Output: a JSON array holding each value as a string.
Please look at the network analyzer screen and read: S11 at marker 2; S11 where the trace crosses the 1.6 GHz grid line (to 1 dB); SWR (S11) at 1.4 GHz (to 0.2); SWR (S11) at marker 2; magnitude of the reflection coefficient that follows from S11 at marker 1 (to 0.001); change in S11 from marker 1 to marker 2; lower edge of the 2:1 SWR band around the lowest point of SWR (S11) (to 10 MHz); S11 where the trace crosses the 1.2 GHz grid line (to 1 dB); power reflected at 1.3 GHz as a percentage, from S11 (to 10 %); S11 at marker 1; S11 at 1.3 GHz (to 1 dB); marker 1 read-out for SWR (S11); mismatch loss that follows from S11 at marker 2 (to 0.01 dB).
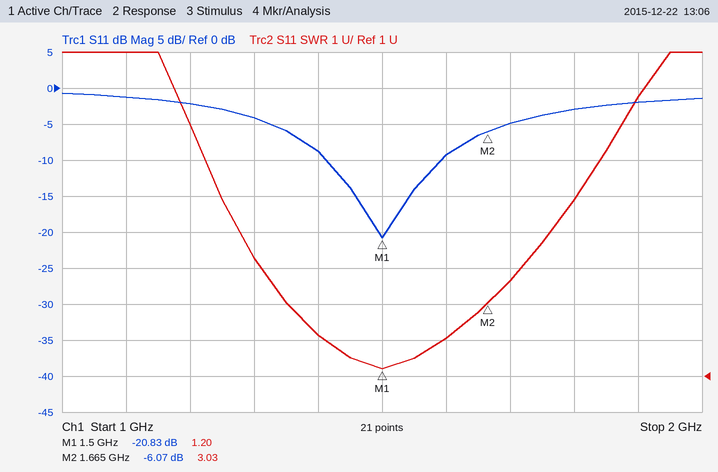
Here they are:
["-6.07 dB", "-9 dB", "2.2", "3.03", "0.091", "14.76 dB", "1.41 GHz", "-2 dB", "40 %", "-20.83 dB", "-4 dB", "1.20", "1.23 dB"]
